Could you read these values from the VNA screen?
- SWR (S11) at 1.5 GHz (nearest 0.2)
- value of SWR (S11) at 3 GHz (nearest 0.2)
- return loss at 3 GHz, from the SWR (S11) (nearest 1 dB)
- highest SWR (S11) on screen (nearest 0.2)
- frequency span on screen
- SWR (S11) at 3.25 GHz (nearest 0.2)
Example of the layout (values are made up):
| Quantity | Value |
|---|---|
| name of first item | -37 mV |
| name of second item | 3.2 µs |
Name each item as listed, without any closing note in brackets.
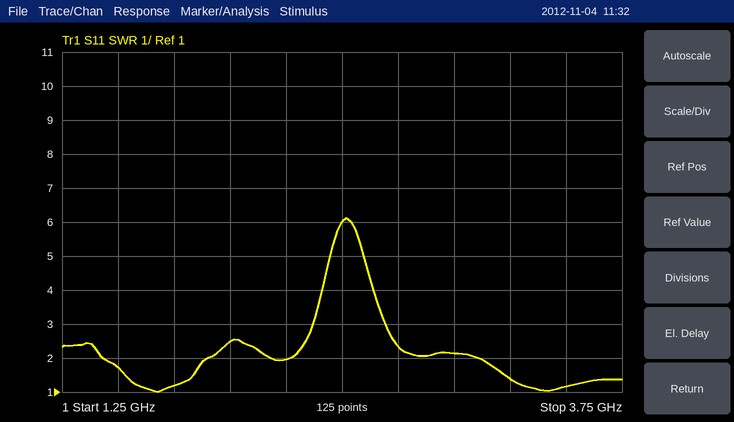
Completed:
| Quantity | Value |
|---|---|
| SWR (S11) at 1.5 GHz | 1.8 |
| value of SWR (S11) at 3 GHz | 2.2 |
| return loss at 3 GHz, from the SWR (S11) | 9 dB |
| highest SWR (S11) on screen | 6.2 |
| frequency span on screen | 2.5 GHz |
| SWR (S11) at 3.25 GHz | 1.4 |
